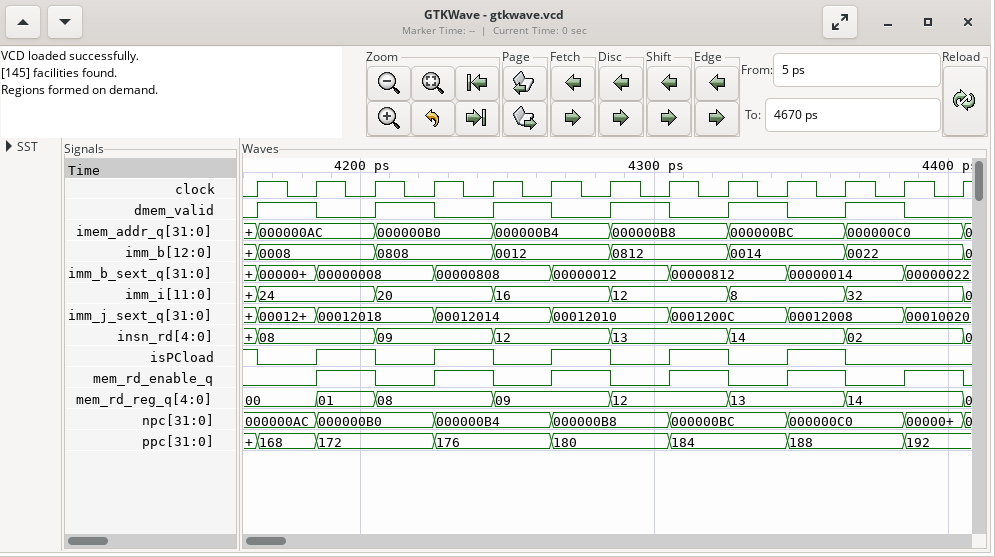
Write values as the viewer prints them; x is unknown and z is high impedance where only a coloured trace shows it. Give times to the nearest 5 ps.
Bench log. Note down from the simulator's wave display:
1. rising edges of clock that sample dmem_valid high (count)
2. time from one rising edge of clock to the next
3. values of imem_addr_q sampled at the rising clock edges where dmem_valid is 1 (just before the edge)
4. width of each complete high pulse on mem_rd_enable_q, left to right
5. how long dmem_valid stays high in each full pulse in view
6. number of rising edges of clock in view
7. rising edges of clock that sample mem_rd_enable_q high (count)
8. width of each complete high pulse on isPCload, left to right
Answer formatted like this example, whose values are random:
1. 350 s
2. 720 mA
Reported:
1. 6
2. 20 ps
3. 000000AC, 000000B0, 000000B4, 000000B8, 000000BC, 000000C0
4. 20 ps, 20 ps, 20 ps, 20 ps, 20 ps, 20 ps
5. 20 ps, 20 ps, 20 ps, 20 ps, 20 ps, 20 ps
6. 13
7. 6
8. 20 ps, 20 ps, 20 ps, 20 ps, 20 ps
